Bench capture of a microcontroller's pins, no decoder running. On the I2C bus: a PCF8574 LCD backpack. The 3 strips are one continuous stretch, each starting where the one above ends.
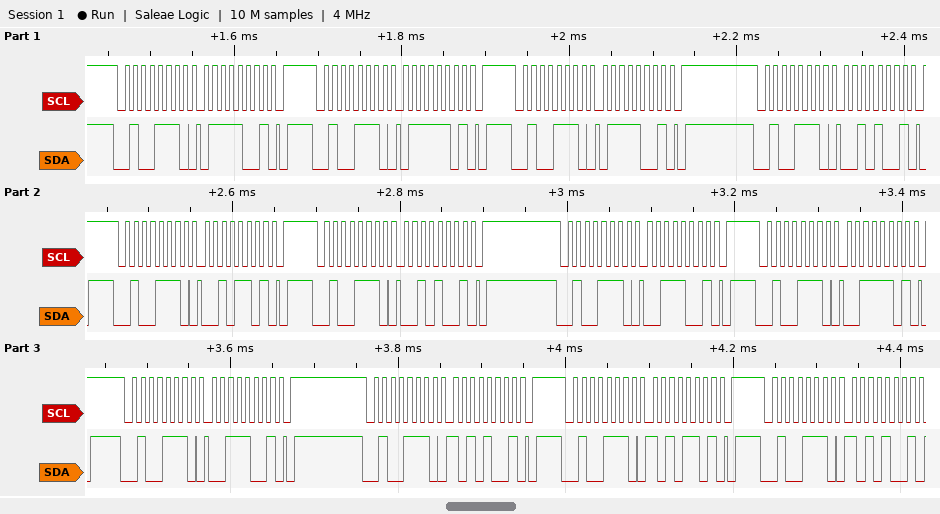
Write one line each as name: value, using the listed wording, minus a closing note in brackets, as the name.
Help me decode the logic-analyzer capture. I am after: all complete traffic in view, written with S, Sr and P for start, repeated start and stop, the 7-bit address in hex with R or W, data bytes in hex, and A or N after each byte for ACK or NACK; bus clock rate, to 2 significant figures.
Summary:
all complete traffic in view, written with S, Sr and P for start, repeated start and stop, the 7-bit address in hex with R or W, data bytes in hex, and A or N after each byte for ACK or NACK: S 27W A 79 A P S 27W A 7D A P S 27W A 79 A P S 27W A 29 A P S 27W A 2D A P S 27W A 29 A P S 27W A 39 A P S 27W A 3D A P S 27W A 39 A P S 27W A A9 A P S 27W A AD A P S 27W A A9 A
bus clock rate, to 2 significant figures: 100 kHz
